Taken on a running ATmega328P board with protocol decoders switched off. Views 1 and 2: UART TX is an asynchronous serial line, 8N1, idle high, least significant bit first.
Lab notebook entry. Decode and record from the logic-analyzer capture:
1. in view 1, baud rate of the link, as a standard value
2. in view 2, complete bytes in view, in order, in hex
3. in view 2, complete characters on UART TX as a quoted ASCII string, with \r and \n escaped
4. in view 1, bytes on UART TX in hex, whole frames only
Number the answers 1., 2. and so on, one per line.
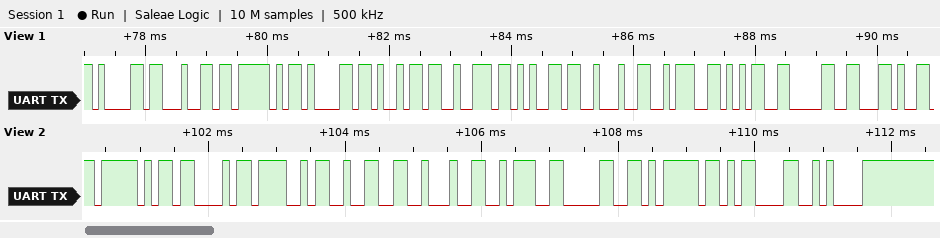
1. 9600 baud
2. 5F 43 4F 32 22 3A 30 7D 0D 0A
3. "_CO2\":0}\r\n"
4. 61 64 5F 61 69 72 65 22 3A 35 30 2C
